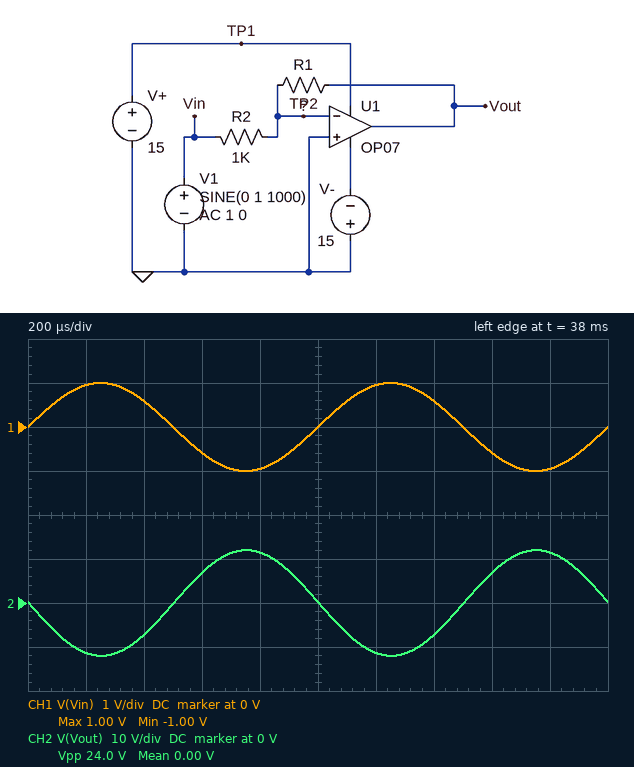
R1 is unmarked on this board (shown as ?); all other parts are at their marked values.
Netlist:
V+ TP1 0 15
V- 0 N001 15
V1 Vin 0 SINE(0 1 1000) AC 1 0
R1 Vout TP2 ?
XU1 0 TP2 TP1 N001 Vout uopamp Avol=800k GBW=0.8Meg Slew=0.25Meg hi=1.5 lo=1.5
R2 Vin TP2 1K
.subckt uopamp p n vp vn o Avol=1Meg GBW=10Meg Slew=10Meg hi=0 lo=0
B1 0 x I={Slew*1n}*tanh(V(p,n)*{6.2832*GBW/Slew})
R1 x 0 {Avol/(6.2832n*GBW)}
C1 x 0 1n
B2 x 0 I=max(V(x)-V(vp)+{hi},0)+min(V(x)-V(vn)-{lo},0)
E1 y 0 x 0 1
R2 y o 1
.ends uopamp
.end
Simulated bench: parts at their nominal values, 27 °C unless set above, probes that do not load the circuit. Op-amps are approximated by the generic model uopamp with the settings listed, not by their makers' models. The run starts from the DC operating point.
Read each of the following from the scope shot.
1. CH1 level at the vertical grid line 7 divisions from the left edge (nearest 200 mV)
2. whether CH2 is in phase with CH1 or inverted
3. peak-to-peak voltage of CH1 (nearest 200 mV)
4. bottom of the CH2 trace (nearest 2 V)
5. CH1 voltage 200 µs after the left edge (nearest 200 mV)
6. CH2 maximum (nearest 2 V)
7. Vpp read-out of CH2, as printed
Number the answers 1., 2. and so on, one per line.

1. 600 mV
2. inverted
3. 2.0 V
4. -12 V
5. 1.0 V
6. 12 V
7. 24.0 V
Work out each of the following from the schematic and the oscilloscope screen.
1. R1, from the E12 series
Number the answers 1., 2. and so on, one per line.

1. 12 kΩ
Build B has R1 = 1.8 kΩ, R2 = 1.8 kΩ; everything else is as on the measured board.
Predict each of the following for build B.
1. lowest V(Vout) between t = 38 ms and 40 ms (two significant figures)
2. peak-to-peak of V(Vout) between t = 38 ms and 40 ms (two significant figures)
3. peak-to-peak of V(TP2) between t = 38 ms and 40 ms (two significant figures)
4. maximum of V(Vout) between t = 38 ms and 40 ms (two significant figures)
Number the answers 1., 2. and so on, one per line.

1. -1.0 V
2. 2.0 V
3. 2.5 mV
4. 1.0 V
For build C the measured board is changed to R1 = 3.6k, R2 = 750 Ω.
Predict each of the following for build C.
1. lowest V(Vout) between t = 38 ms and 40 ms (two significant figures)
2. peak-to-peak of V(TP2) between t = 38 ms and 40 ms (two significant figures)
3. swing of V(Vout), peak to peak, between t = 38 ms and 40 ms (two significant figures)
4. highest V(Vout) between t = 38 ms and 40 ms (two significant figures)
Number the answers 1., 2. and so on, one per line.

1. -4.8 V
2. 12 mV
3. 9.6 V
4. 4.8 V
